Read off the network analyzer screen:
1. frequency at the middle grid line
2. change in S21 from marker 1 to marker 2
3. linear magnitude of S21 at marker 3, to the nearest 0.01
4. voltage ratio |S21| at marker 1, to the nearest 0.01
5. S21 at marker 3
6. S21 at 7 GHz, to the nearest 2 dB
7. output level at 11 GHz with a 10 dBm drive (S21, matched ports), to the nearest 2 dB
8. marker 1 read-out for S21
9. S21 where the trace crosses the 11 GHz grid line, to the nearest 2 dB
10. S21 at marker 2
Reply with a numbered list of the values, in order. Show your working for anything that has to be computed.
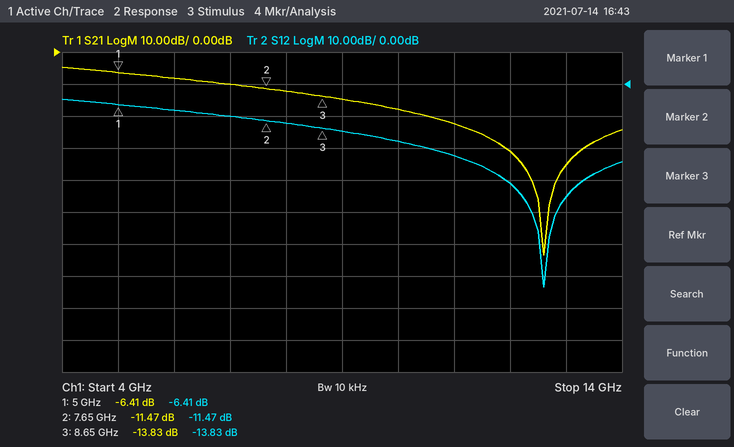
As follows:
1. 9 GHz
2. -11.47 − (-6.41) = -5.06 dB
3. 10^(-13.83/20) ≈ 0.20
4. 10^(-6.41/20) ≈ 0.48
5. -13.83 dB
6. -10 dB
7. 10 dBm + (-22 dB) = -12 dBm
8. -6.41 dB
9. -22 dB
10. -11.47 dB
